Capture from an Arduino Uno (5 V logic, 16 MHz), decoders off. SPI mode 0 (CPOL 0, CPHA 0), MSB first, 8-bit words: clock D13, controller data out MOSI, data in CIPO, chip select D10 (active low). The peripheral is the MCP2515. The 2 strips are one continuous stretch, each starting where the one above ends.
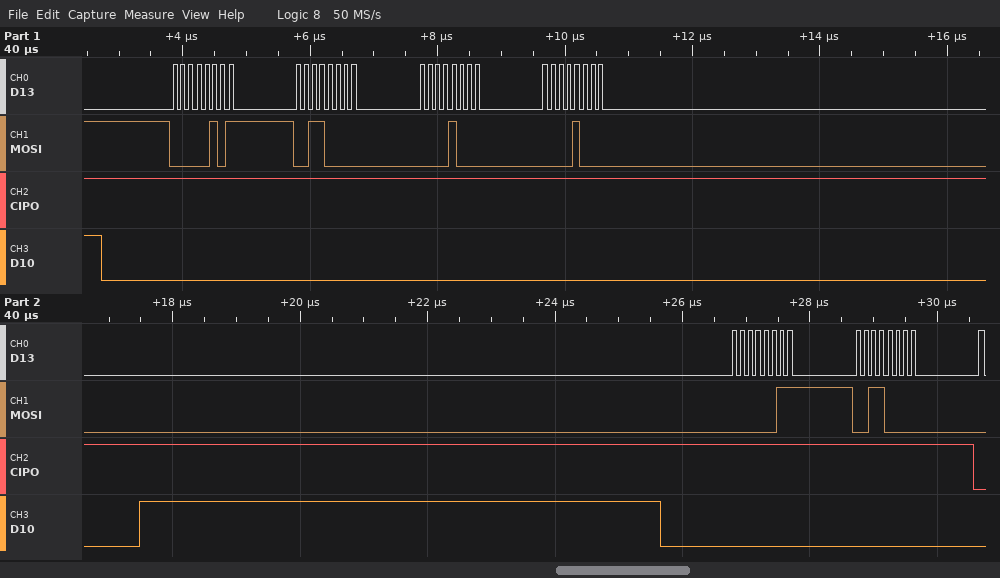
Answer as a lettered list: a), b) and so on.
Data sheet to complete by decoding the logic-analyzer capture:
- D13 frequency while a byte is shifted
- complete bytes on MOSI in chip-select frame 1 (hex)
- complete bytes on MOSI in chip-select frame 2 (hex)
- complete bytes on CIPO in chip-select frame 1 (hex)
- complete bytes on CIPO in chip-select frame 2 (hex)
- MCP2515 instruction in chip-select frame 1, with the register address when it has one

a) 8 MHz
b) 05 30 08 08
c) 03 30
d) FF FF FF FF
e) FF FF
f) BIT MODIFY 0x30
